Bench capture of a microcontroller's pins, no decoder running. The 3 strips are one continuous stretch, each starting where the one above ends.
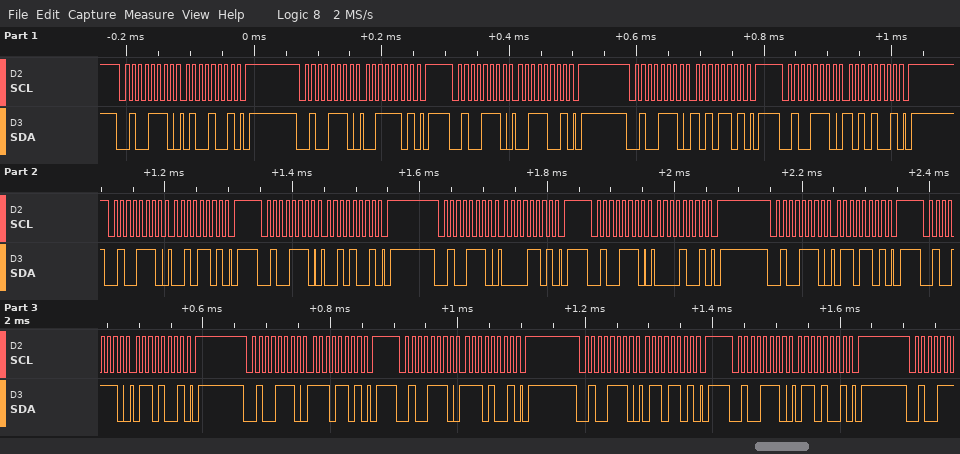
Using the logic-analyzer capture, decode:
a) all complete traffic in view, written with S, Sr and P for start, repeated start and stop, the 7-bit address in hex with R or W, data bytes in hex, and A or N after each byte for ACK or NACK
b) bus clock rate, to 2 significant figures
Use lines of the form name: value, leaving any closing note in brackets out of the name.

all complete traffic in view, written with S, Sr and P for start, repeated start and stop, the 7-bit address in hex with R or W, data bytes in hex, and A or N after each byte for ACK or NACK: S 27W A 49 A P S 27W A 3D A P S 27W A 39 A P S 27W A AD A P S 27W A A9 A P S 27W A 2D A P S 27W A 29 A P S 27W A 0D A P S 27W A 09 A P S 27W A 6D A P S 27W A 69 A P S 27W A ED A P S 27W A E9 A P S 27W A 6D A P S 27W A 69 A P
bus clock rate, to 2 significant figures: 100 kHz
